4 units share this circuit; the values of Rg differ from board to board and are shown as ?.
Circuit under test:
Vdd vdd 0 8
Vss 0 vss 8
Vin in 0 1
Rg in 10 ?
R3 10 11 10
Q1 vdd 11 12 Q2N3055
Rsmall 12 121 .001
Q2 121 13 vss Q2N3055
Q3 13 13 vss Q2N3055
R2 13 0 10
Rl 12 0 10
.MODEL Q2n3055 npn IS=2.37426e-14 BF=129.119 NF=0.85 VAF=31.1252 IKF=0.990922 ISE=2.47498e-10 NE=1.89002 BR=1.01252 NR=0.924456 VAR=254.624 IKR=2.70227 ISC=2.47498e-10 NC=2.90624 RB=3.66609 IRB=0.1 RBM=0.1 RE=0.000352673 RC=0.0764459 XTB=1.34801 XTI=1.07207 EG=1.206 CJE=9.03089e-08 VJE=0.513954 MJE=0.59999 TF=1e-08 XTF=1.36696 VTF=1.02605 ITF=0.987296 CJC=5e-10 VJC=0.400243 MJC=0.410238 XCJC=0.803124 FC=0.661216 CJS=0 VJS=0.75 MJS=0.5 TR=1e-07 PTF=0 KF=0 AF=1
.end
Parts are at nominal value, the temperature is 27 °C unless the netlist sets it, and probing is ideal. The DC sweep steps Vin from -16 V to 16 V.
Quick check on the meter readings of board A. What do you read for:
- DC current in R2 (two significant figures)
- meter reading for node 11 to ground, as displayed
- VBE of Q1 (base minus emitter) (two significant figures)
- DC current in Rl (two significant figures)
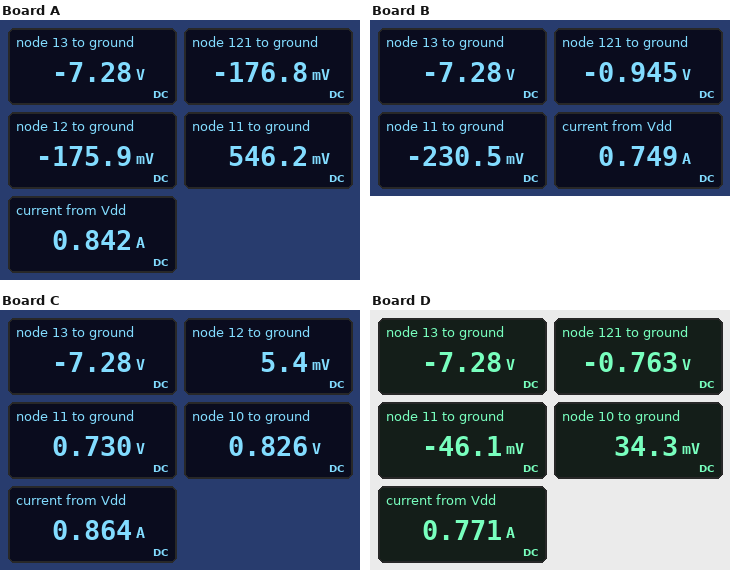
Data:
730 mA
546.2 mV
720 mV
18 mA
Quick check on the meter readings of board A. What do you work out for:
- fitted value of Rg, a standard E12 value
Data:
39 Ω
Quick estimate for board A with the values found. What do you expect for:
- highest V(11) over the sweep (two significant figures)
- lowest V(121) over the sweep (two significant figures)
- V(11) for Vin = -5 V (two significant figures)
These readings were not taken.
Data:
8.8 V
-7.1 V
-5.1 V
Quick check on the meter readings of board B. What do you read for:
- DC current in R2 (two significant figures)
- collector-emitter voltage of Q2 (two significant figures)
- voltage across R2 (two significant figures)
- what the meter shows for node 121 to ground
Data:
730 mA
7.1 V
7.3 V
-0.945 V
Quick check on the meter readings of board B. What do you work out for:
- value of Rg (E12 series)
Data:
150 Ω
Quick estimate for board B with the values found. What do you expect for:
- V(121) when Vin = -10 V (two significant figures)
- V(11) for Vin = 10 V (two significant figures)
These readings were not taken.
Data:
-7.1 V
5.8 V
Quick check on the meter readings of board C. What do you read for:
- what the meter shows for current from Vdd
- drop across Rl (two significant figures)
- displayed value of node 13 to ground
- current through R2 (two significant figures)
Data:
0.864 A
5.4 mV
-7.28 V
730 mA
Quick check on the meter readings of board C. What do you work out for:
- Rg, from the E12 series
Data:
18 Ω
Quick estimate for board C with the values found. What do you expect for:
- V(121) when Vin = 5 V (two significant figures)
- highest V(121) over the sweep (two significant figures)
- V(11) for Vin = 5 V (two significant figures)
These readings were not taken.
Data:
3.7 V
7.9 V
4.4 V
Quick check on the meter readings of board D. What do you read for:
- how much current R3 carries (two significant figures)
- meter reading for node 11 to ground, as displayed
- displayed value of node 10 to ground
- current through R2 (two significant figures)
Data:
8.0 mA
-46.1 mV
34.3 mV
730 mA
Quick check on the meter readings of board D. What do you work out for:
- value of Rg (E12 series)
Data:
120 Ω
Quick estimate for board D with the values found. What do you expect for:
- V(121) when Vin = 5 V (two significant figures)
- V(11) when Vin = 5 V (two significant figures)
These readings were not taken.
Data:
2.2 V
3.0 V
